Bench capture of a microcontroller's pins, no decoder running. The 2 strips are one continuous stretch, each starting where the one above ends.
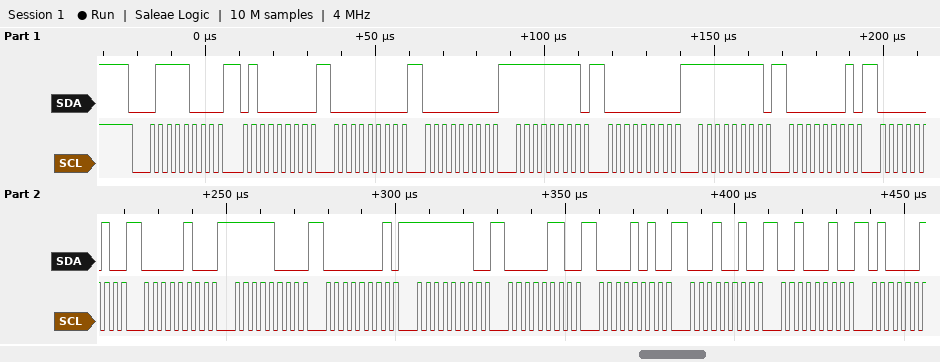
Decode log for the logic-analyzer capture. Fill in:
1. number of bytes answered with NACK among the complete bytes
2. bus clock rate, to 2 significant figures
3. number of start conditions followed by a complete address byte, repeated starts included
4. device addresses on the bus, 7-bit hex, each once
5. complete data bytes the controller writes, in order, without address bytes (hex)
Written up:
0
400 kHz
1
0x3C
40 00 00 FF 00 FF 01 02 04 F8 01 FE 06 0A 12 22
